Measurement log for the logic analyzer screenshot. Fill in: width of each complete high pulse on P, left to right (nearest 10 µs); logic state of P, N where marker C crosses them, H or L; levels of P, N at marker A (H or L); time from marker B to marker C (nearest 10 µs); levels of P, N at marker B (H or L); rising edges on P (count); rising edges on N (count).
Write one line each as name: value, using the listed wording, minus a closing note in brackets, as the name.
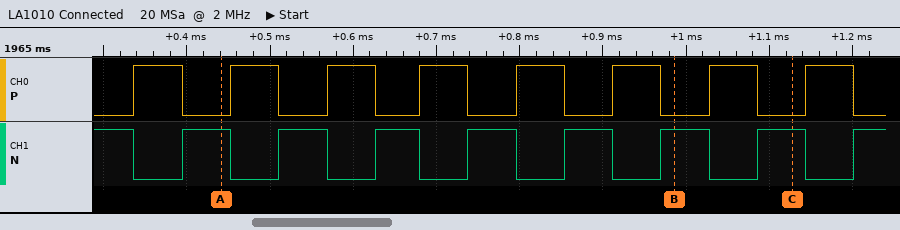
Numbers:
width of each complete high pulse on P, left to right: 60 µs, 60 µs, 60 µs, 60 µs, 60 µs, 60 µs, 60 µs, 60 µs
logic state of P, N where marker C crosses them, H or L: P=L, N=H
levels of P, N at marker A: P=L, N=H
time from marker B to marker C: 140 µs
levels of P, N at marker B: P=L, N=H
rising edges on P: 8
rising edges on N: 8
